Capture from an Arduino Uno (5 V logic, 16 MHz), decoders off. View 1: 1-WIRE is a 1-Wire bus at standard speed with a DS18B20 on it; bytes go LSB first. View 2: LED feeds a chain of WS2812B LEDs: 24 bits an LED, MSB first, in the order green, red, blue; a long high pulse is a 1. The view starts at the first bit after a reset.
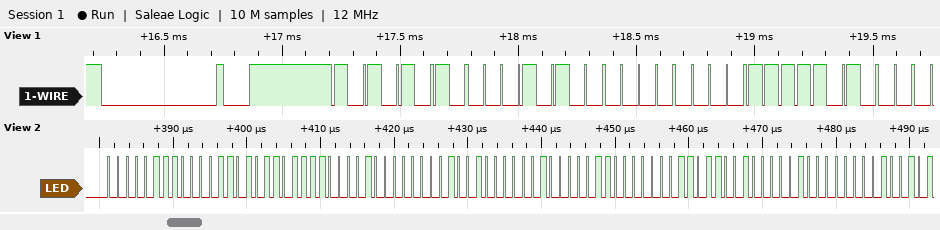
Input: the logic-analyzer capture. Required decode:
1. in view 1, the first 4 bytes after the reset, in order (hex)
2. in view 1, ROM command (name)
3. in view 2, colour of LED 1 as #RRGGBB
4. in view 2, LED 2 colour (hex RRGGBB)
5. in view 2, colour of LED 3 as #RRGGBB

55 28 00 5F
Match ROM
#0D076F
#040881
#030664
